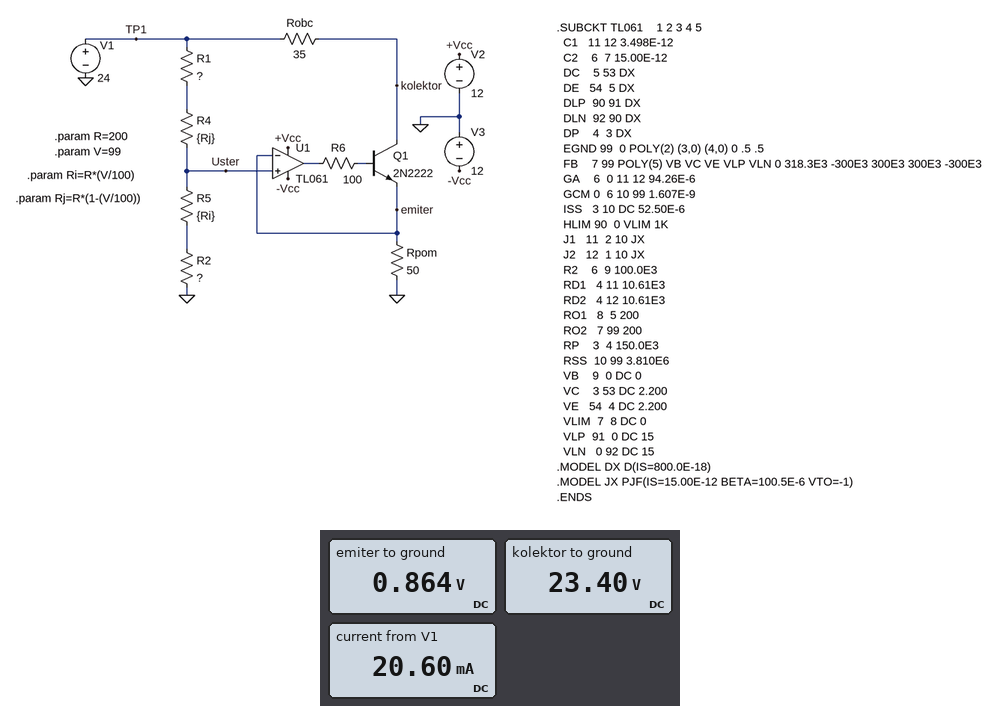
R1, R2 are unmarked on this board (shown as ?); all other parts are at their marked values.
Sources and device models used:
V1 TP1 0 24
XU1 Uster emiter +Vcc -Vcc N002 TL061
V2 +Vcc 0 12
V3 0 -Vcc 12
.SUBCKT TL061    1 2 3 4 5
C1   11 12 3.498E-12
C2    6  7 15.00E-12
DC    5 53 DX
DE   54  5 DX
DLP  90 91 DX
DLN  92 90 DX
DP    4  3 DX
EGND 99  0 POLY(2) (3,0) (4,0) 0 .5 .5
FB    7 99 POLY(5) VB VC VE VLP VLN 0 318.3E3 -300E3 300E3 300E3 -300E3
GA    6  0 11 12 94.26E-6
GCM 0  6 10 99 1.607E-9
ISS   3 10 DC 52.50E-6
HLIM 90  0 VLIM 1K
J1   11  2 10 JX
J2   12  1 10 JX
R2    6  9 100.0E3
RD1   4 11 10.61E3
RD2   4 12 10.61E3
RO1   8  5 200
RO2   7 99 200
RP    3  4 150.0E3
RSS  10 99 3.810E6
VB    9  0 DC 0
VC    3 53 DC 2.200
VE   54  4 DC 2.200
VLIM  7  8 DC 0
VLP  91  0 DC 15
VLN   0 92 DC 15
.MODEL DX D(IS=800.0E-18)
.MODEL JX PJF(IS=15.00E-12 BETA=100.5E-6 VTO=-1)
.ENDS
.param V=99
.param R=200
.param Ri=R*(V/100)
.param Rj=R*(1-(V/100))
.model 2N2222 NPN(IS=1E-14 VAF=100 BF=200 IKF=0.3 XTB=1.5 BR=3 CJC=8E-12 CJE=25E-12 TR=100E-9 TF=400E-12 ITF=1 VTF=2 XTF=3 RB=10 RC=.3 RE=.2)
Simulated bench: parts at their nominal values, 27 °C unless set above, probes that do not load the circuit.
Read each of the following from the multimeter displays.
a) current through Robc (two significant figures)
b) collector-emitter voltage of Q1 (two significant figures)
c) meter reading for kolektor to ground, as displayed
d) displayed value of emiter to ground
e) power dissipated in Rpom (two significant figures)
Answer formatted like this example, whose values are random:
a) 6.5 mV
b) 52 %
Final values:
a) 17 mA
b) 23 V
c) 23.40 V
d) 0.864 V
e) 15 mW
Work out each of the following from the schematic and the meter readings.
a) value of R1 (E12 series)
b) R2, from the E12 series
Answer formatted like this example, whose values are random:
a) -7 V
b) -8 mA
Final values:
a) 6.8 kΩ
b) 56 Ω
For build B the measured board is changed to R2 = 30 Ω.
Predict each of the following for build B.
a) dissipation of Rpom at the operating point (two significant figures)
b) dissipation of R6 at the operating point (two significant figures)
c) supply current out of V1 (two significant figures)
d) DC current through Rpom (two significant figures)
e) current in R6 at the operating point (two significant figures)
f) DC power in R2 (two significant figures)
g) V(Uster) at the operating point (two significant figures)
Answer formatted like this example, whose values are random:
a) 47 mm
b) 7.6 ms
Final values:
a) 12 mW
b) 440 nW
c) 19 mA
d) 16 mA
e) 66 µA
f) 350 µW
g) 780 mV
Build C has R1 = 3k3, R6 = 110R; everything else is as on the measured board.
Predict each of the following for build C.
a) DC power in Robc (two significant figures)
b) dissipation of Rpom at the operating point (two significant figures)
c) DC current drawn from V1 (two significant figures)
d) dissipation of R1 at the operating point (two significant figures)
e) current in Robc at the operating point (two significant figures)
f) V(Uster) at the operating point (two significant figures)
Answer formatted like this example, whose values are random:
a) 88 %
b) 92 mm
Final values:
a) 41 mW
b) 59 mW
c) 41 mA
d) 150 mW
e) 34 mA
f) 1.7 V
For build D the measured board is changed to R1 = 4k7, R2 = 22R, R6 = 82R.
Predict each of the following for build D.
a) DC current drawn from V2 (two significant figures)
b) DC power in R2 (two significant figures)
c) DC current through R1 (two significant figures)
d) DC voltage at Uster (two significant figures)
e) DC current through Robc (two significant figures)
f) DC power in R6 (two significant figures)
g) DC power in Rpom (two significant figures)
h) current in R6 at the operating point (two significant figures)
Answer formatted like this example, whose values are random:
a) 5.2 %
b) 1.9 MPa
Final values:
a) 210 µA
b) 520 µW
c) 4.9 mA
d) 1.1 V
e) 21 mA
f) 710 nW
g) 23 mW
h) 93 µA
